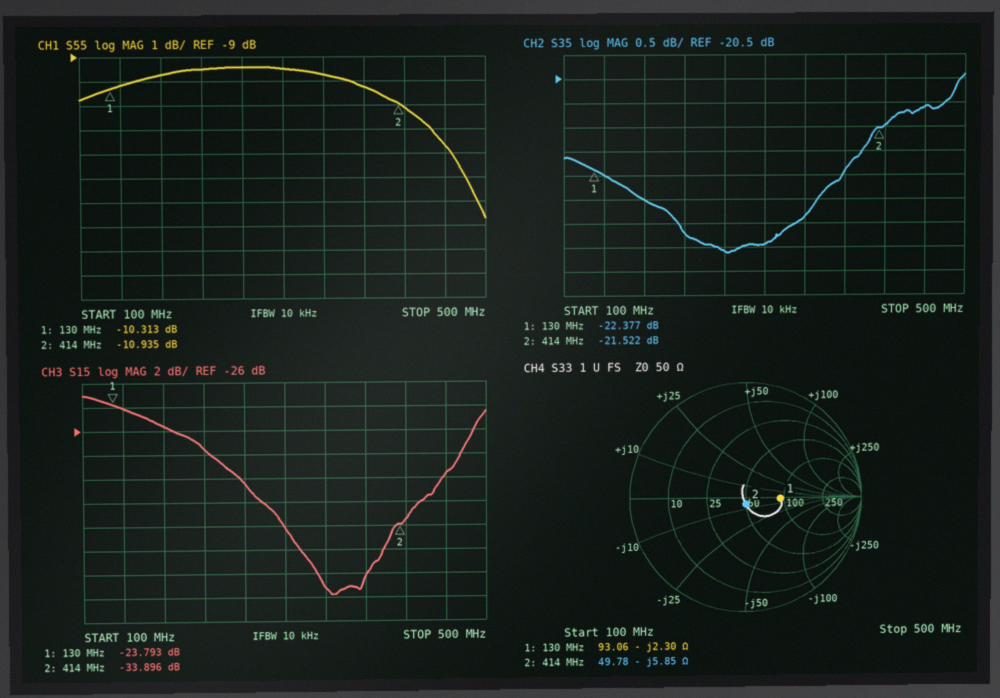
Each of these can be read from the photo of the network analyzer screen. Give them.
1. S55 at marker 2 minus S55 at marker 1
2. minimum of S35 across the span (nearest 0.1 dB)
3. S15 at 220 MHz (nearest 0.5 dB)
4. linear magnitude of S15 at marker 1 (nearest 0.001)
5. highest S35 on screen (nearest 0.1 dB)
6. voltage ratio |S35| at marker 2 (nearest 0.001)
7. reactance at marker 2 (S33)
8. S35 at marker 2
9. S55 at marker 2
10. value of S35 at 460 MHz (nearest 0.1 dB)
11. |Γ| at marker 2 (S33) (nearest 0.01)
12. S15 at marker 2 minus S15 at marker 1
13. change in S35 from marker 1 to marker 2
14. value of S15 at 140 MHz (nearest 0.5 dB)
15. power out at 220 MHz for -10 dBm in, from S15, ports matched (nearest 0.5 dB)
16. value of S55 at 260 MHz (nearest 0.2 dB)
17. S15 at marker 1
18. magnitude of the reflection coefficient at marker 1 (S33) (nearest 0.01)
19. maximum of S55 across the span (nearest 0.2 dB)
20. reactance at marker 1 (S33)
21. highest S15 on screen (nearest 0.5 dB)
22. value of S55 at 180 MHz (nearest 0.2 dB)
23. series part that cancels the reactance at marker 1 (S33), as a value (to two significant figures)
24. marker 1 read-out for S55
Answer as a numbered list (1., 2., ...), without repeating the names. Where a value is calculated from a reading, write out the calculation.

1. -10.935 − (-10.313) = -0.622 dB
2. -24.1 dB
3. -27.5 dB
4. 10^(-23.793/20) ≈ 0.065
5. -20.4 dB
6. 10^(-21.522/20) ≈ 0.084
7. -5.85 Ω
8. -21.522 dB
9. -10.935 dB
10. -21.1 dB
11. 0.06
12. -33.896 − (-23.793) = -10.103 dB
13. -21.522 − (-22.377) = 0.855 dB
14. -24.0 dB
15. -10 dBm + (-27.5 dB) = -37.5 dBm
16. -9.4 dB
17. -23.793 dB
18. 0.30
19. -9.4 dB
20. -2.30 Ω
21. -23.0 dB
22. -9.8 dB
23. L = 2.3 Ω/(2π × 130 MHz) ≈ 2.8 nH
24. -10.313 dB
